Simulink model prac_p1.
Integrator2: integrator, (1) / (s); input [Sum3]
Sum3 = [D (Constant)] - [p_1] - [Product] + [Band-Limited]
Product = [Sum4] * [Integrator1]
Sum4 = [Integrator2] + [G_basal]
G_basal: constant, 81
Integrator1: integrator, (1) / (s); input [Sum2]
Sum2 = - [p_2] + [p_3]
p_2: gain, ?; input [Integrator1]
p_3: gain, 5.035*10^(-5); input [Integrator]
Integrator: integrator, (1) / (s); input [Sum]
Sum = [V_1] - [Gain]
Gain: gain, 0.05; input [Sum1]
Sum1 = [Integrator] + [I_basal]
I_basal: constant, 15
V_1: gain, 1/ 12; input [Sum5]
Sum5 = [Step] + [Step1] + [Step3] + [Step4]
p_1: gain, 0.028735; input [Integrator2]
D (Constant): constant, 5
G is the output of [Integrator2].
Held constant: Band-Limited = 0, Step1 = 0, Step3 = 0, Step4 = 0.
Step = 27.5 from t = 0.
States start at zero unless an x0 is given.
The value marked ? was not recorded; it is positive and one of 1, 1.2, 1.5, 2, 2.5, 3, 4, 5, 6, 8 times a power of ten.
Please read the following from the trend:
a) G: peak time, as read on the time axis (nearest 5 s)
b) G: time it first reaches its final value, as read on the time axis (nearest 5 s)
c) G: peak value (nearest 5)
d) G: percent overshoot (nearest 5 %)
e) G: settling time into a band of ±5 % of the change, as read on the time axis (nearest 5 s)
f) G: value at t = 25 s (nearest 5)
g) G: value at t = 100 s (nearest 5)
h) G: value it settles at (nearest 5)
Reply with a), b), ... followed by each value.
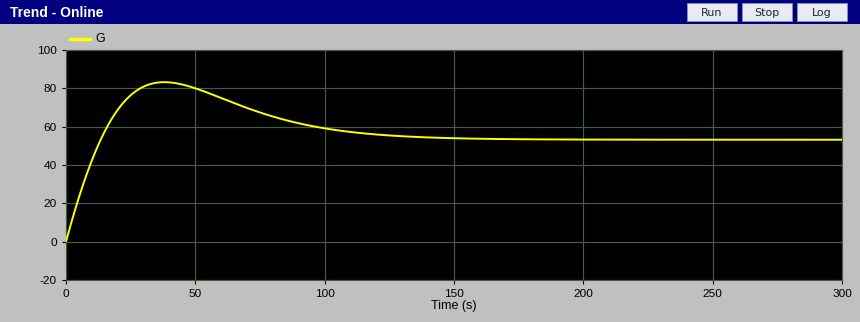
a) 40 s
b) 15 s
c) 85
d) 55 %
e) 120 s
f) 75
g) 60
h) 55
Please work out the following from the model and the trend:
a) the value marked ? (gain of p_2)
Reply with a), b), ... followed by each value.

a) 0.06
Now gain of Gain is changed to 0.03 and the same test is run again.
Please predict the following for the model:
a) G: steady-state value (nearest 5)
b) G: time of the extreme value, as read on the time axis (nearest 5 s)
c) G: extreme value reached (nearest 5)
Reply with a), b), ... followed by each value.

a) 10
b) 30 s
c) 75
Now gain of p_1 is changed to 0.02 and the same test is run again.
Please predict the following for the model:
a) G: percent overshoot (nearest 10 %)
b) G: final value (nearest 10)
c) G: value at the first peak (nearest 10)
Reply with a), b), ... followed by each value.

a) 50 %
b) 60
c) 100
